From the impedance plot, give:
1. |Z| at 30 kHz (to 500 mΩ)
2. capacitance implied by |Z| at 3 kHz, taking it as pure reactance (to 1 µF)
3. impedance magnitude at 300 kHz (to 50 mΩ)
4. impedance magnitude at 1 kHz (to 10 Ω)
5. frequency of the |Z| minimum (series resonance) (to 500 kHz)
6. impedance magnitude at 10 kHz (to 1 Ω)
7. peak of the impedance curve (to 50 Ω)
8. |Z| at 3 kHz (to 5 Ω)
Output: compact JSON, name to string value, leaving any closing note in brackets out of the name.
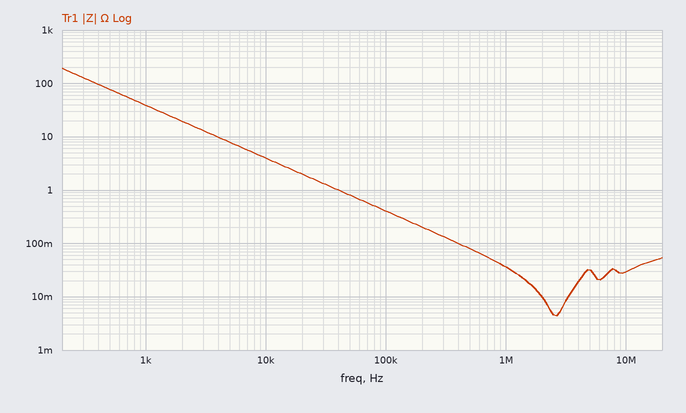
{"|Z| at 30 kHz": "1.5 Ω", "capacitance implied by |Z| at 3 kHz, taking it as pure reactance": "4 µF", "impedance magnitude at 300 kHz": "150 mΩ", "impedance magnitude at 1 kHz": "40 Ω", "frequency of the |Z| minimum (series resonance)": "2.5 MHz", "impedance magnitude at 10 kHz": "4 Ω", "peak of the impedance curve": "200 Ω", "|Z| at 3 kHz": "15 Ω"}
